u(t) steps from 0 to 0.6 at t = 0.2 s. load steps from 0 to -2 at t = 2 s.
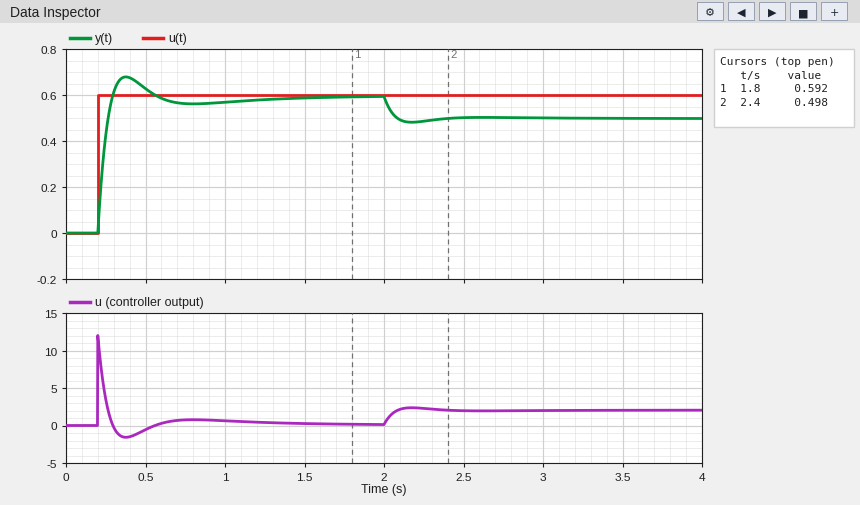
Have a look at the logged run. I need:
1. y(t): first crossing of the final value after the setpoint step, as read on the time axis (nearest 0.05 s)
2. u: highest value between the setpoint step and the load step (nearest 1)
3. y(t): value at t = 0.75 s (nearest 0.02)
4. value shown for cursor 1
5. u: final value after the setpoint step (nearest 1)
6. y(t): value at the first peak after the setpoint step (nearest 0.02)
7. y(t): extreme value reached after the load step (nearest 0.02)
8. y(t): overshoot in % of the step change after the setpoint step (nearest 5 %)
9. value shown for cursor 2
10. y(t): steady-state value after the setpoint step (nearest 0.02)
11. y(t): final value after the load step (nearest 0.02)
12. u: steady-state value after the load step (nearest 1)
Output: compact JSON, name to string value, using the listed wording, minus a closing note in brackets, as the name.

{"y(t): first crossing of the final value after the setpoint step, as read on the time axis": "0.30 s", "u: highest value between the setpoint step and the load step": "12", "y(t): value at t = 0.75 s": "0.56", "value shown for cursor 1": "0.592", "u: final value after the setpoint step": "0", "y(t): value at the first peak after the setpoint step": "0.68", "y(t): extreme value reached after the load step": "0.48", "y(t): overshoot in % of the step change after the setpoint step": "15 %", "value shown for cursor 2": "0.498", "y(t): steady-state value after the setpoint step": "0.60", "y(t): final value after the load step": "0.50", "u: steady-state value after the load step": "2"}
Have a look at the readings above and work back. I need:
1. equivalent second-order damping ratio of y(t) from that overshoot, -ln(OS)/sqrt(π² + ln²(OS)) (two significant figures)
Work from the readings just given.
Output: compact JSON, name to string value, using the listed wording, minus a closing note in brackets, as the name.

{"equivalent second-order damping ratio of y(t) from that overshoot, -ln(OS)/sqrt(π² + ln²(OS))": "0.52"}
